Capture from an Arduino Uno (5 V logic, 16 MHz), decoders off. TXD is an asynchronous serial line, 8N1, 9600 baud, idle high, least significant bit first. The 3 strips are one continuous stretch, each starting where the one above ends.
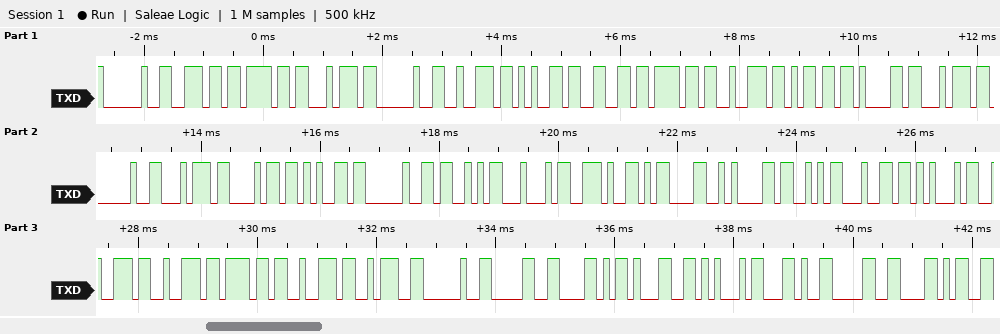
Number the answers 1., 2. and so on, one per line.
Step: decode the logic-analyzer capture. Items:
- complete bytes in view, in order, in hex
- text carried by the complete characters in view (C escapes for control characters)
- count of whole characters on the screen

1. 20 6E 6F 74 20 72 65 66 6F 72 6D 61 74 20 74 68 65 20 53 44 2E 0D 0A 53 64 45 72 72 6F 72 3A 20 30 58 31 45 2C 30 58
2. " not reformat the SD.\r\nSdError: 0X1E,0X"
3. 39
